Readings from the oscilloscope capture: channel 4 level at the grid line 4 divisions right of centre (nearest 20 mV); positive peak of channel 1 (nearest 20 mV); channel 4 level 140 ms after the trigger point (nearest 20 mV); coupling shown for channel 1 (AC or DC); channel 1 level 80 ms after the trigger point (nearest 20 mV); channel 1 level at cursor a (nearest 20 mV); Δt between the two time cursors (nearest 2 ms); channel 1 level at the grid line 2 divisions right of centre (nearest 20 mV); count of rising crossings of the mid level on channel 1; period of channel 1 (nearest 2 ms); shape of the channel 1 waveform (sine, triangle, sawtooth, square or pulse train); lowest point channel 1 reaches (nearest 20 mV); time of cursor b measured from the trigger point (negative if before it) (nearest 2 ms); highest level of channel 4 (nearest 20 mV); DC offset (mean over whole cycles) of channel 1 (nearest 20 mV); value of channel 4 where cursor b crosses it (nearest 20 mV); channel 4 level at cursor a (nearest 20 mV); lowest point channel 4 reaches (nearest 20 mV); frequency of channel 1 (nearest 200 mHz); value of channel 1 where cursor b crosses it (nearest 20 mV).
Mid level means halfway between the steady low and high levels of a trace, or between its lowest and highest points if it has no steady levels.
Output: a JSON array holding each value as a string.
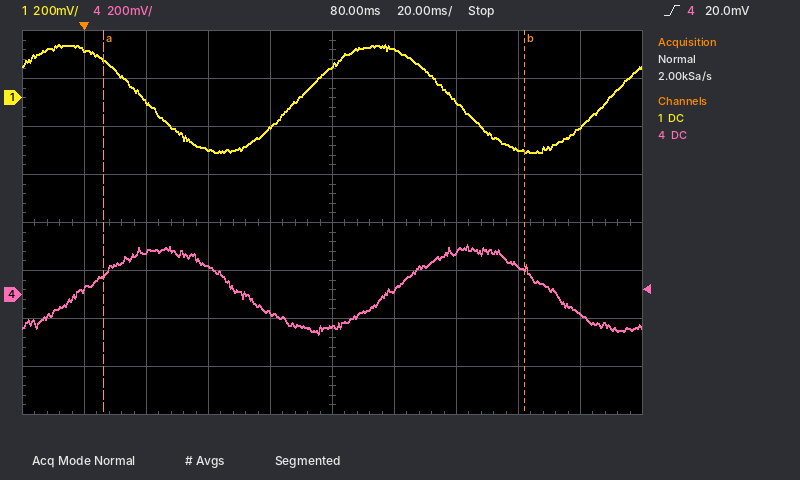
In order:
["-80 mV", "220 mV", "120 mV", "DC", "140 mV", "160 mV", "136 ms", "-20 mV", "2", "100 ms", "sine", "-220 mV", "+142 ms", "200 mV", "0 mV", "100 mV", "80 mV", "-160 mV", "10.0 Hz", "-220 mV"]
